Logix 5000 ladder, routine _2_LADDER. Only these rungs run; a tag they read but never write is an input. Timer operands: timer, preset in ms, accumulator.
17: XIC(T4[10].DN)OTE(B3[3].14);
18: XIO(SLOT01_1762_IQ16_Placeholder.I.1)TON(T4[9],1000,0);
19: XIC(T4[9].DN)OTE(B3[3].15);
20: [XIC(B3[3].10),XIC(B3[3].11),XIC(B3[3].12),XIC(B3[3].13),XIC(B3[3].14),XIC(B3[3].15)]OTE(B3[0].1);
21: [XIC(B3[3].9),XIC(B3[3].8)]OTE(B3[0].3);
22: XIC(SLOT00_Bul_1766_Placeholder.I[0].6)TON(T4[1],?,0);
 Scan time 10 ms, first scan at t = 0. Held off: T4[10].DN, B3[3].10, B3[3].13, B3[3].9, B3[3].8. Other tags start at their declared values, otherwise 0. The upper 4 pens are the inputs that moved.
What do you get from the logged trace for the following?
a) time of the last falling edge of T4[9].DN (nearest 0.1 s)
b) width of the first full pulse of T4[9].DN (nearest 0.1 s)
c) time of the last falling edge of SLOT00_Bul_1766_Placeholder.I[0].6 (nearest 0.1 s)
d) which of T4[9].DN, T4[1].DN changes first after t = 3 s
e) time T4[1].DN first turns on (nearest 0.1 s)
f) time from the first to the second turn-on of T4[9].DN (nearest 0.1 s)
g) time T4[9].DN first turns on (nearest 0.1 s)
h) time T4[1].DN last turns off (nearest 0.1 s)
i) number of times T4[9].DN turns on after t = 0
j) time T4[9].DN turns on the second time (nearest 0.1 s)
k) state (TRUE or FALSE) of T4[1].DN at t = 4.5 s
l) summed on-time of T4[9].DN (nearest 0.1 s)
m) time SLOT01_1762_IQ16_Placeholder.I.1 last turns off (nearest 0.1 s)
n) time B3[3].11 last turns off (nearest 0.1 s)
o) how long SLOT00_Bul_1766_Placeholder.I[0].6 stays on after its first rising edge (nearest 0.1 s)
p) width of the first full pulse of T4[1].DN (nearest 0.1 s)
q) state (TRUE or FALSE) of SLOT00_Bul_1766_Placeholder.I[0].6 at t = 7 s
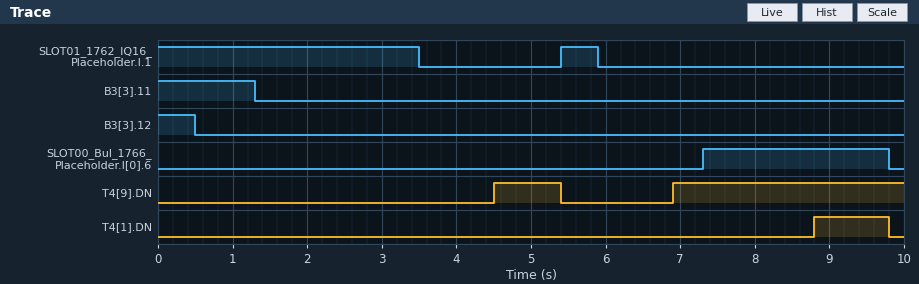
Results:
5.4 s
0.9 s
9.8 s
T4[9].DN
8.8 s
2.4 s
4.5 s
9.8 s
2
6.9 s
FALSE
4.0 s
5.9 s
1.3 s
2.5 s
1.0 s
FALSE
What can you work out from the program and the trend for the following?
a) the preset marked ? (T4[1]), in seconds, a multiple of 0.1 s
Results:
1.5 s
